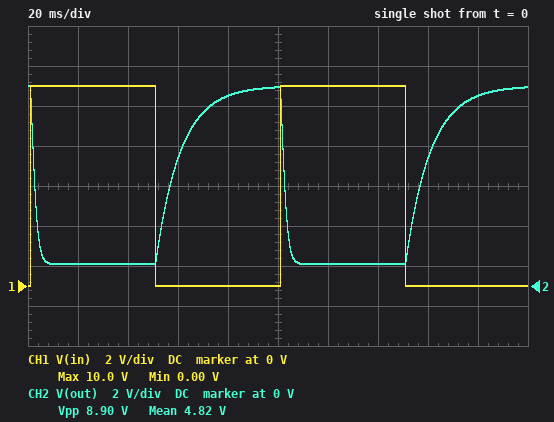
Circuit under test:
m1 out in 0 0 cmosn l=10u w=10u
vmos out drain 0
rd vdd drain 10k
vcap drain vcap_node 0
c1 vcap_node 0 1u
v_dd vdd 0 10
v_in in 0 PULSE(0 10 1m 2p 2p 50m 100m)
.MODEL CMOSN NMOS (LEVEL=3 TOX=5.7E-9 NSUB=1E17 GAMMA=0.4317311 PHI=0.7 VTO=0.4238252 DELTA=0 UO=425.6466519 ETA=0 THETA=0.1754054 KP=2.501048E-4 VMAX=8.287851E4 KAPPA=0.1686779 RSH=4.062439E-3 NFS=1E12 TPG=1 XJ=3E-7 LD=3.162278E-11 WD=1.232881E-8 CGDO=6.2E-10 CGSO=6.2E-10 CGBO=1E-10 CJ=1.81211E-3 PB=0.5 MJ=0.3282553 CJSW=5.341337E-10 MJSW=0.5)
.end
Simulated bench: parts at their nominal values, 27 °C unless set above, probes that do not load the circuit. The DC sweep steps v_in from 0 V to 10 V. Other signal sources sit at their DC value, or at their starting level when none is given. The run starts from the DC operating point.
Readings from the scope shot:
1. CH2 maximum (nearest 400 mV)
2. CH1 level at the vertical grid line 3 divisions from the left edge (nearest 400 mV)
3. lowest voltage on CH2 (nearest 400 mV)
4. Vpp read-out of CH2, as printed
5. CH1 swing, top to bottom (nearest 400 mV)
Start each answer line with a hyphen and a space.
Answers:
- 10.0 V
- 0 V
- 1.2 V
- 8.90 V
- 10.0 V
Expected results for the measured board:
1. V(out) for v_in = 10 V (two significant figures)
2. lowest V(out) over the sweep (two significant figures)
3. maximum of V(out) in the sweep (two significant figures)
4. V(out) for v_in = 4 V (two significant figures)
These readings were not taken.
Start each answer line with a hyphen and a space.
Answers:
- 1.1 V
- 1.1 V
- 10 V
- 2.4 V
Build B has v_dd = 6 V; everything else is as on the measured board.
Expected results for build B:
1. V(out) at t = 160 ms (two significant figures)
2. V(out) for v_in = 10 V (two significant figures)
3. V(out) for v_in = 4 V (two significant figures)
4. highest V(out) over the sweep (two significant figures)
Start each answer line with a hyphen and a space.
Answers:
- 3.8 V
- 630 mV
- 1.1 V
- 6.0 V
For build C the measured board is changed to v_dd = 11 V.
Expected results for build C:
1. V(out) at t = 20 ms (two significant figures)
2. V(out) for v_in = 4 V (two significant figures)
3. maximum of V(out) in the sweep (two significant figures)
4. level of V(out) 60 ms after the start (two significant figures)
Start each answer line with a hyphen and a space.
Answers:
- 1.2 V
- 3.1 V
- 11 V
- 7.0 V
